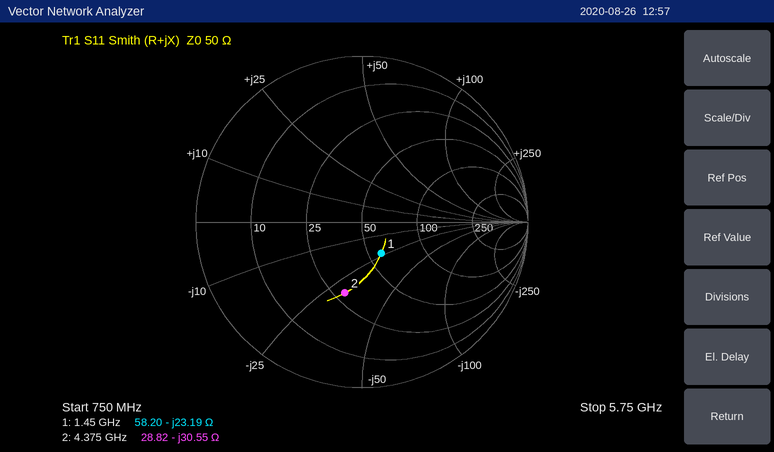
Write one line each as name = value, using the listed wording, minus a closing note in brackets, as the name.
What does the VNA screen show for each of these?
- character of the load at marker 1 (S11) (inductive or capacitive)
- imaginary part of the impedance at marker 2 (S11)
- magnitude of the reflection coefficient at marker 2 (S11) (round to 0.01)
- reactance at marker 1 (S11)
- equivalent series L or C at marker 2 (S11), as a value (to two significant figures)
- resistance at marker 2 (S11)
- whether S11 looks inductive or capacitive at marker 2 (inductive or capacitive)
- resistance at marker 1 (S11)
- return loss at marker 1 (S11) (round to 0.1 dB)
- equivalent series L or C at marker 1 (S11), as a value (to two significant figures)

character of the load at marker 1 (S11) = capacitive
imaginary part of the impedance at marker 2 = -30.55 Ω
magnitude of the reflection coefficient at marker 2 (S11) = 0.44
reactance at marker 1 = -23.19 Ω
equivalent series L or C at marker 2 (S11), as a value = 1.2 pF
resistance at marker 2 = 28.82 Ω
whether S11 looks inductive or capacitive at marker 2 = capacitive
resistance at marker 1 = 58.20 Ω
return loss at marker 1 (S11) = 13.1 dB
equivalent series L or C at marker 1 (S11), as a value = 4.7 pF
